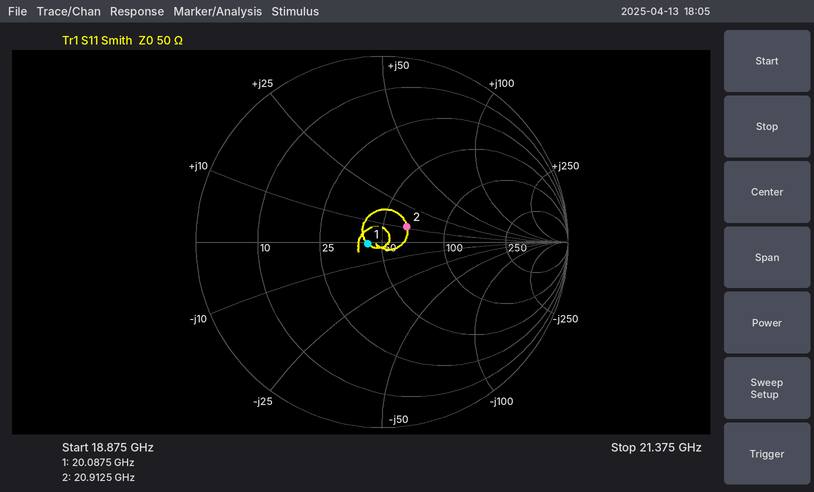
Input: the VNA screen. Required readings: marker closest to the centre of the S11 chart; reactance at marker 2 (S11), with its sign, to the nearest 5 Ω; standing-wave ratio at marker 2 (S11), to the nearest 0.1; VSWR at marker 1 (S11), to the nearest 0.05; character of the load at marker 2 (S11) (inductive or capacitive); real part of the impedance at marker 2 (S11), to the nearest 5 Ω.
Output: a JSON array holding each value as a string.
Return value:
["marker 1", "+10 Ω", "1.4", "1.15", "inductive", "65 Ω"]
